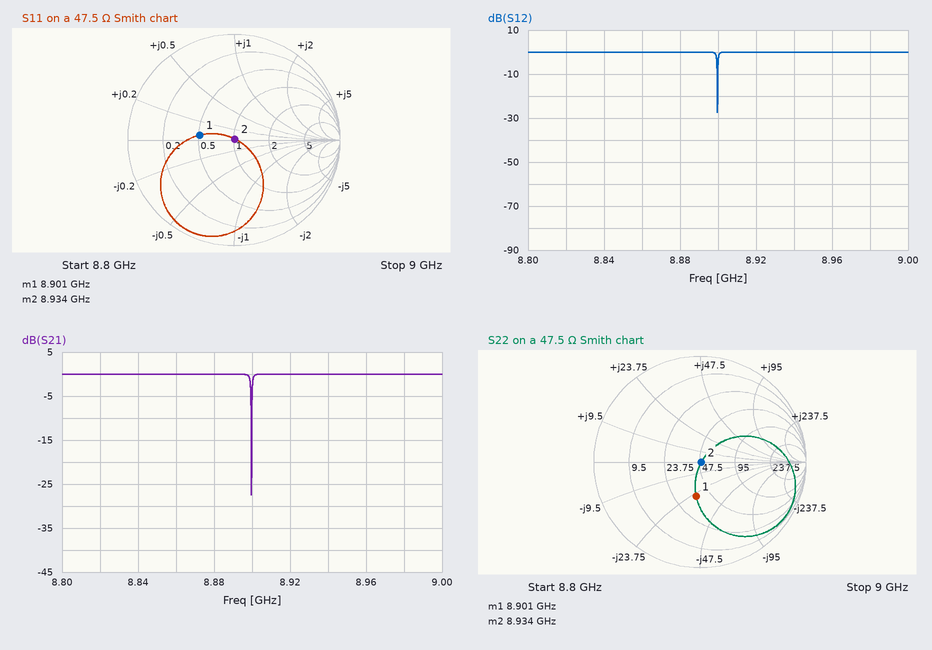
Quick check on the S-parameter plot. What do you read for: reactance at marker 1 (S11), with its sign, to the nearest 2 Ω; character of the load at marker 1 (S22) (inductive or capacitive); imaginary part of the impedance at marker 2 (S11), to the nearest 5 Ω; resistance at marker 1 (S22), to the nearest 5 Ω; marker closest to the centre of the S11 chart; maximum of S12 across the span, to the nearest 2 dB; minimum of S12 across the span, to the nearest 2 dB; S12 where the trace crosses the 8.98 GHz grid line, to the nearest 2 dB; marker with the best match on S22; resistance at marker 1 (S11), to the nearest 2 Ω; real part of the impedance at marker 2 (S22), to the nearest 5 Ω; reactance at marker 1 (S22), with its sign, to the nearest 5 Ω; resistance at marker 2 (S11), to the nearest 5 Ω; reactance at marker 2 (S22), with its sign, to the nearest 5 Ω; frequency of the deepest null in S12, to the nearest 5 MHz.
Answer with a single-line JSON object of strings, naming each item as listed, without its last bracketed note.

{"reactance at marker 1 (S11), with its sign, to the nearest 2 Ω": "+2 Ω", "character of the load at marker 1 (S22)": "capacitive", "imaginary part of the impedance at marker 2 (S11), to the nearest 5 Ω": "0 Ω", "resistance at marker 1 (S22), to the nearest 5 Ω": "35 Ω", "marker closest to the centre of the S11 chart": "marker 2", "maximum of S12 across the span, to the nearest 2 dB": "0 dB", "minimum of S12 across the span, to the nearest 2 dB": "-28 dB", "S12 where the trace crosses the 8.98 GHz grid line, to the nearest 2 dB": "0 dB", "marker with the best match on S22": "marker 2", "resistance at marker 1 (S11), to the nearest 2 Ω": "24 Ω", "real part of the impedance at marker 2 (S22), to the nearest 5 Ω": "50 Ω", "reactance at marker 1 (S22), with its sign, to the nearest 5 Ω": "-25 Ω", "resistance at marker 2 (S11), to the nearest 5 Ω": "50 Ω", "reactance at marker 2 (S22), with its sign, to the nearest 5 Ω": "0 Ω", "frequency of the deepest null in S12, to the nearest 5 MHz": "8.900 GHz"}
